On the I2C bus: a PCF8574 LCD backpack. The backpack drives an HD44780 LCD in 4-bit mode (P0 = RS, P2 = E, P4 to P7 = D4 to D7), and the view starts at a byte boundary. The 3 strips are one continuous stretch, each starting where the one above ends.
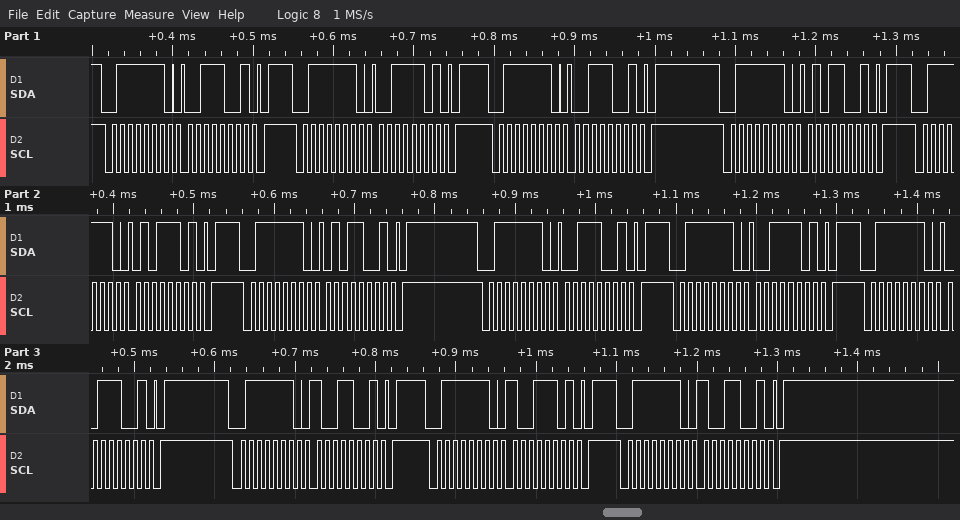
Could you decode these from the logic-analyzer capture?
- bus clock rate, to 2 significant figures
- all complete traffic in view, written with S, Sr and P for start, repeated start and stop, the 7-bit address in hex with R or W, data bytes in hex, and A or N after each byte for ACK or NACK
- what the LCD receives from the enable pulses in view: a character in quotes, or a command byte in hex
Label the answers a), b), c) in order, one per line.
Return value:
a) 100 kHz
b) S 3FW A 39 A P S 3FW A 3D A P S 3FW A 39 A P S 3FW A 59 A P S 3FW A 5D A P S 3FW A 59 A P S 3FW A 39 A P S 3FW A 3D A P S 3FW A 39 A P S 3FW A 99 A P S 3FW A 9D A P S 3FW A 99 A P
c) '5' '9'
